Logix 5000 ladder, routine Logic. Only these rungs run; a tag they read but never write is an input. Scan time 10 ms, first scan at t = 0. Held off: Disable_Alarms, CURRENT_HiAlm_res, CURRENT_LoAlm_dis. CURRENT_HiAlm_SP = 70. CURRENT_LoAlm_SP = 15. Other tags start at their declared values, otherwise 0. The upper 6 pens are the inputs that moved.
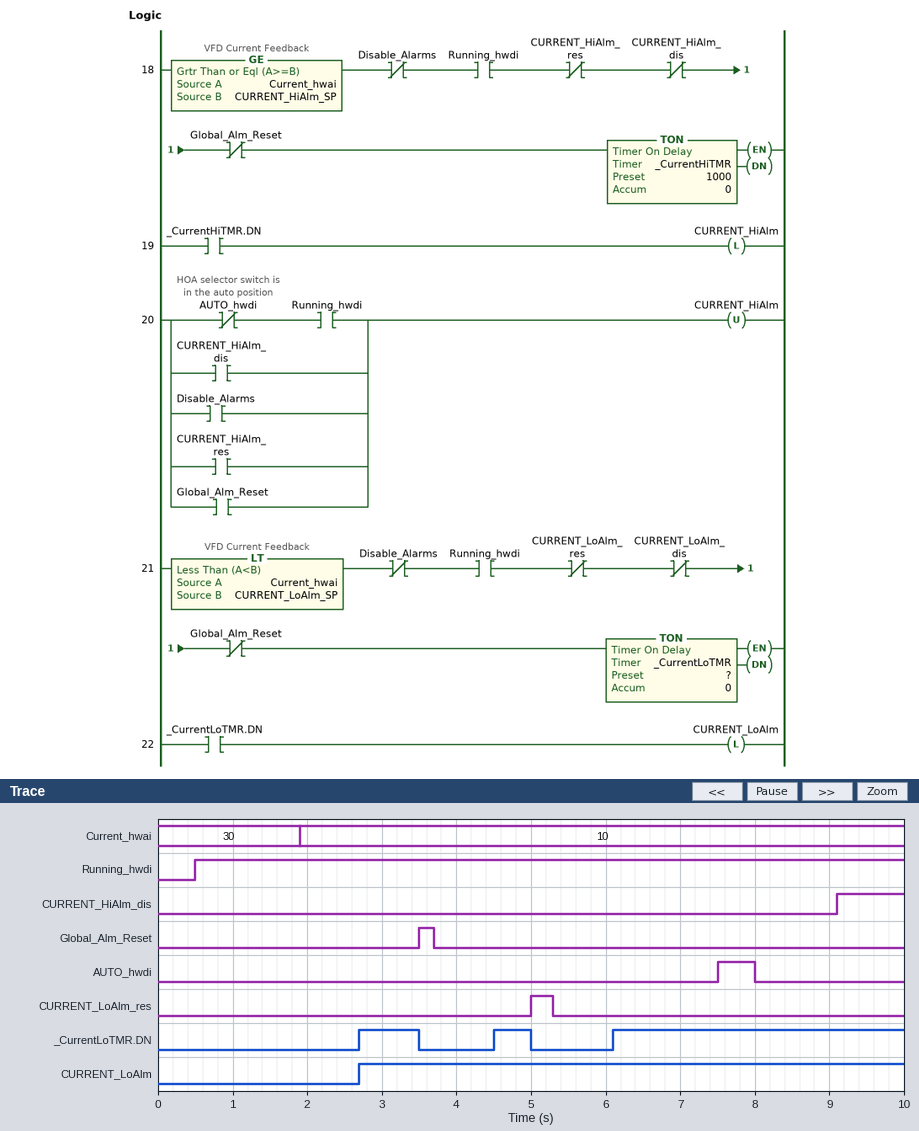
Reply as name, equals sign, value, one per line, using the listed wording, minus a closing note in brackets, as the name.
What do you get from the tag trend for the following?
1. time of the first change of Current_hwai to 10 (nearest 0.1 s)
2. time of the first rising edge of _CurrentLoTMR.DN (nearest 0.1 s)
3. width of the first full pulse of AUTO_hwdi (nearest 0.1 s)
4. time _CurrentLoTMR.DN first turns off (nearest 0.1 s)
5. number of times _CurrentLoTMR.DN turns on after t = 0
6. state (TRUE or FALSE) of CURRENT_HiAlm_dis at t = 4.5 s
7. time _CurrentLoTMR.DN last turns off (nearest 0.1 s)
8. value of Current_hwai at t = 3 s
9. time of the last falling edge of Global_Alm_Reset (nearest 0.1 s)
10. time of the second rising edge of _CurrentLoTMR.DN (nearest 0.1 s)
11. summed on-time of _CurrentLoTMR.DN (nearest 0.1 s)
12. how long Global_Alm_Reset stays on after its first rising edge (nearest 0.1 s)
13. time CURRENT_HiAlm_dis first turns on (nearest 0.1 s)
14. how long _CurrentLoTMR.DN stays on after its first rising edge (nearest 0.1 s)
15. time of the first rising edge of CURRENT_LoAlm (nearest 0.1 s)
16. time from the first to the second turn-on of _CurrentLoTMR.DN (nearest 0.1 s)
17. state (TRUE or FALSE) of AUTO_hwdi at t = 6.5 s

time of the first change of Current_hwai to 10 = 1.9 s
time of the first rising edge of _CurrentLoTMR.DN = 2.7 s
width of the first full pulse of AUTO_hwdi = 0.5 s
time _CurrentLoTMR.DN first turns off = 3.5 s
number of times _CurrentLoTMR.DN turns on after t = 0 = 3
state (TRUE or FALSE) of CURRENT_HiAlm_dis at t = 4.5 s = FALSE
time _CurrentLoTMR.DN last turns off = 5.0 s
value of Current_hwai at t = 3 s = 10
time of the last falling edge of Global_Alm_Reset = 3.7 s
time of the second rising edge of _CurrentLoTMR.DN = 4.5 s
summed on-time of _CurrentLoTMR.DN = 5.2 s
how long Global_Alm_Reset stays on after its first rising edge = 0.2 s
time CURRENT_HiAlm_dis first turns on = 9.1 s
how long _CurrentLoTMR.DN stays on after its first rising edge = 0.8 s
time of the first rising edge of CURRENT_LoAlm = 2.7 s
time from the first to the second turn-on of _CurrentLoTMR.DN = 1.8 s
state (TRUE or FALSE) of AUTO_hwdi at t = 6.5 s = FALSE
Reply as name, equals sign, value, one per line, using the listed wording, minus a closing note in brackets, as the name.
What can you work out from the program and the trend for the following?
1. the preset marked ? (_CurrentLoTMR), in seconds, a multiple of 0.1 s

the preset marked ? (_CurrentLoTMR), in seconds, a multiple of 0.1 s = 0.8 s
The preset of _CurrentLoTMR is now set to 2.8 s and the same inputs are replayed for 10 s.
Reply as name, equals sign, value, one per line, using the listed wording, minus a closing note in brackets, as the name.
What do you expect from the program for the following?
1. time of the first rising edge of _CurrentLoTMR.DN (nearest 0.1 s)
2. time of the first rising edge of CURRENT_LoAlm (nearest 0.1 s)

time of the first rising edge of _CurrentLoTMR.DN = 8.1 s
time of the first rising edge of CURRENT_LoAlm = 8.1 s
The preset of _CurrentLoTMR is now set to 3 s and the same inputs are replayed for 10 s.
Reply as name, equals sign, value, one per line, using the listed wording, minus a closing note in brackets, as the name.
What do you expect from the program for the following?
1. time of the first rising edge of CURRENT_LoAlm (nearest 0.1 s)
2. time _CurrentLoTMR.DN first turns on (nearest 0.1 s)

time of the first rising edge of CURRENT_LoAlm = 8.3 s
time _CurrentLoTMR.DN first turns on = 8.3 s
